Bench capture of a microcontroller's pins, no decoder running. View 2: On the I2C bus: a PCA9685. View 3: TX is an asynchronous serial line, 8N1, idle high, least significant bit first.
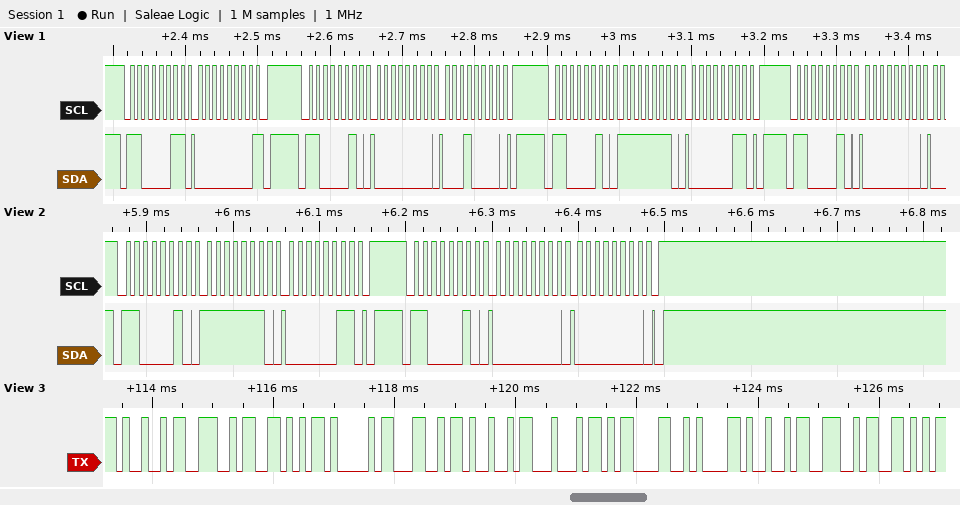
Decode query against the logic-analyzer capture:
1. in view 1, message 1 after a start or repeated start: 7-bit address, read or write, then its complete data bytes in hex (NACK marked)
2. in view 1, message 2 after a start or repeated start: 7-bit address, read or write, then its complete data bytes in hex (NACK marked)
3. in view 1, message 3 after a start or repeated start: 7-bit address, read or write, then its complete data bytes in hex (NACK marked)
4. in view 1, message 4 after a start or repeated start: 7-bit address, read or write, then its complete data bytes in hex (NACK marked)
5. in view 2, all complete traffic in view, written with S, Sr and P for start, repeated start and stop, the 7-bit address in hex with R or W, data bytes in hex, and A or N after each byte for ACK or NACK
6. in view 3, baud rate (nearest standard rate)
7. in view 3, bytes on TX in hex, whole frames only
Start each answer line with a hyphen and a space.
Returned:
- 0x61 read: 00 NACK
- 0x61 write: 00 10
- 0x61 write: FE 03
- 0x61 write: 00
- S 61W A FE A 03 A P S 61W A 00 A 00 A P
- 9600 baud
- 49 4E 56 41 4C 49 44 0D 0A 49 4E 56
